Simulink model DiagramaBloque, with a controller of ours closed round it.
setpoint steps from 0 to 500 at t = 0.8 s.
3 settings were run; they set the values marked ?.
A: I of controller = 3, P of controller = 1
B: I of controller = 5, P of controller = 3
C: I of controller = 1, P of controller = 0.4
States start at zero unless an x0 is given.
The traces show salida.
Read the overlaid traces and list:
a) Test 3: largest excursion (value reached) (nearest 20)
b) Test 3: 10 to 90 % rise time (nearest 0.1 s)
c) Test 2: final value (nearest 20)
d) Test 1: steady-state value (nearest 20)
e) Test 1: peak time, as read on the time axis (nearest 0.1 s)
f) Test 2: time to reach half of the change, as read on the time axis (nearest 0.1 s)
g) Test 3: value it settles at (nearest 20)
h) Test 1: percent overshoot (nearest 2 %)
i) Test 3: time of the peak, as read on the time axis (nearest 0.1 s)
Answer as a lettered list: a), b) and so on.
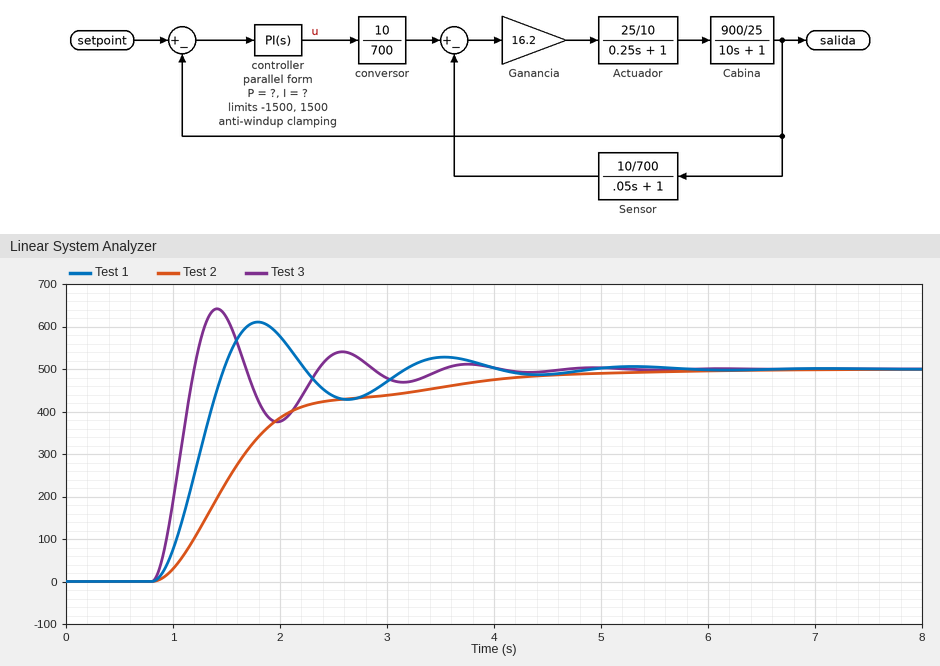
a) 640
b) 0.3 s
c) 500
d) 500
e) 1.8 s
f) 1.5 s
g) 500
h) 22 %
i) 1.4 s
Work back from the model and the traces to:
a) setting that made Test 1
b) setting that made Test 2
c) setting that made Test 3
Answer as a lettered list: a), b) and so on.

a) A
b) C
c) B
